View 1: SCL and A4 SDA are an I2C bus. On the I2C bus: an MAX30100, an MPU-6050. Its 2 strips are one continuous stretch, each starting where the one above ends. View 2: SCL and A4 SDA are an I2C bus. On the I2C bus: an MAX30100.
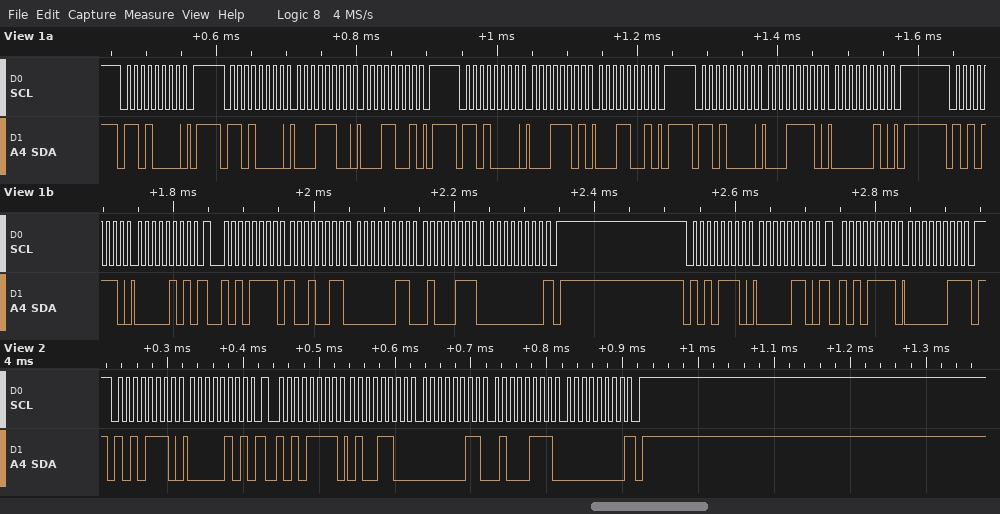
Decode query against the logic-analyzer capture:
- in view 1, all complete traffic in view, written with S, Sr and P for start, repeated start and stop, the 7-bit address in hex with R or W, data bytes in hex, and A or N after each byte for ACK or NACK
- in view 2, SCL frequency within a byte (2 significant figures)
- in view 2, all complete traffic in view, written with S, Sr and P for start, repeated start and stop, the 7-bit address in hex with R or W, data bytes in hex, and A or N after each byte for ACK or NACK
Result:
S 68W A P S 68W A 1C A 19 A P S 68W A 1D A 19 A P S 68W A 1E A 02 A P S 57W A 05 A Sr 57R A 93 A 03 A 47 A 00 N P S 57W A 06 A Sr 57R A 03 N P
100 kHz
S 57W A 05 A Sr 57R A 4C A 03 A 47 A 00 N P
